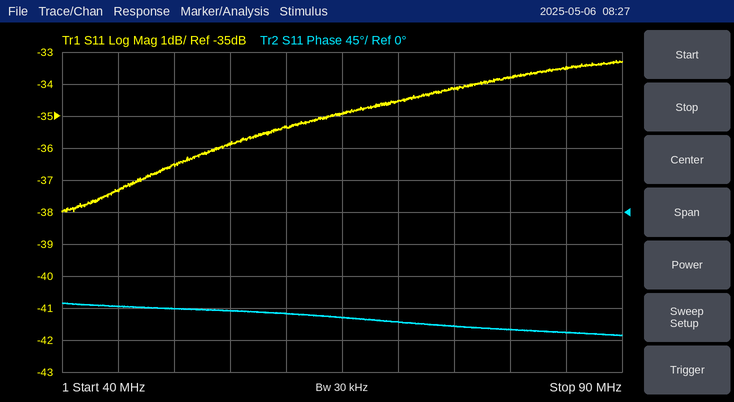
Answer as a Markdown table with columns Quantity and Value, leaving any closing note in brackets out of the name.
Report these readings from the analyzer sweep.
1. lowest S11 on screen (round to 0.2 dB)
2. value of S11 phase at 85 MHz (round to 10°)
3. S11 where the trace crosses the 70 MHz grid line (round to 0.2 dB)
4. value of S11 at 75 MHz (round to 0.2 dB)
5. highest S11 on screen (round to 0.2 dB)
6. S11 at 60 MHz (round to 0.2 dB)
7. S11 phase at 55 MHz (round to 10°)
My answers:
| Quantity | Value |
|---|---|
| lowest S11 on screen | -38.0 dB |
| value of S11 phase at 85 MHz | -170° |
| S11 where the trace crosses the 70 MHz grid line | -34.6 dB |
| value of S11 at 75 MHz | -34.2 dB |
| highest S11 on screen | -33.2 dB |
| S11 at 60 MHz | -35.4 dB |
| S11 phase at 55 MHz | -140° |
